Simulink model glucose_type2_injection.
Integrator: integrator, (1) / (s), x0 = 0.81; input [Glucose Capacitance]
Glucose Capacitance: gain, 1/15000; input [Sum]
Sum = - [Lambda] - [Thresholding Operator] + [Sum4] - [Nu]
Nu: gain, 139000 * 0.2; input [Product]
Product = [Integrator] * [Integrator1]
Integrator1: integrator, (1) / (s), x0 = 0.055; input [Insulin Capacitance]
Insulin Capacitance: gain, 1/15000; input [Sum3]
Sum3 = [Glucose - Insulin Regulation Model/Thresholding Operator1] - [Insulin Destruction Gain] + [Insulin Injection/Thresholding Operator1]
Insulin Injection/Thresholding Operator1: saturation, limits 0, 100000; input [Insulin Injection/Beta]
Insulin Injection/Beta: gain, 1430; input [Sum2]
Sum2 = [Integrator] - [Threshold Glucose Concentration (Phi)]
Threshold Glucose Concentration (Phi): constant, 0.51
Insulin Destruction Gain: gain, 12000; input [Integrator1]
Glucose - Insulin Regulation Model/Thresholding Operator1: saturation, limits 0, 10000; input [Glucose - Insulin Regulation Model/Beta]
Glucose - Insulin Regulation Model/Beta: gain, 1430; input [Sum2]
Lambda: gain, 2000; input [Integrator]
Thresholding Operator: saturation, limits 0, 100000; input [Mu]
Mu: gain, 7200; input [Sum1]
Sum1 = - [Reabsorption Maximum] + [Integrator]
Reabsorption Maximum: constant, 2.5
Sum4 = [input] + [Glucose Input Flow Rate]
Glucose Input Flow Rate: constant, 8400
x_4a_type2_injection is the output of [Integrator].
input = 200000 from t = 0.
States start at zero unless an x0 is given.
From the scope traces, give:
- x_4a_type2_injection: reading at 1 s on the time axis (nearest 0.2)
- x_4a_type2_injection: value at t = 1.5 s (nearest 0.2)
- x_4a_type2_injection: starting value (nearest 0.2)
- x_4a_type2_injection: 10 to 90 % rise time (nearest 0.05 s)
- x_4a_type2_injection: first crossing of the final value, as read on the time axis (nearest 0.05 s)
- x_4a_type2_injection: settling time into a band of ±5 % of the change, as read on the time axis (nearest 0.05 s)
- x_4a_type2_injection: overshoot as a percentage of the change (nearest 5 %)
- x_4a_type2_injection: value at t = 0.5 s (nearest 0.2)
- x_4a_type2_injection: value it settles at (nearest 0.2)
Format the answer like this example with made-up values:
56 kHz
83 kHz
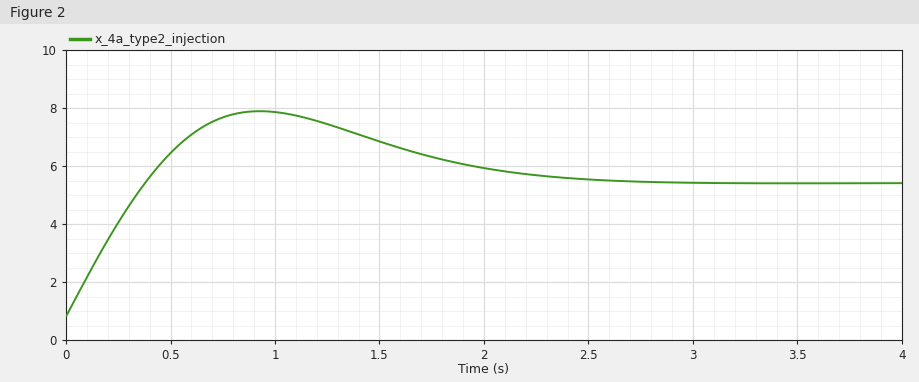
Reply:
7.8
6.8
0.8
0.30 s
0.40 s
2.30 s
55 %
6.4
5.4
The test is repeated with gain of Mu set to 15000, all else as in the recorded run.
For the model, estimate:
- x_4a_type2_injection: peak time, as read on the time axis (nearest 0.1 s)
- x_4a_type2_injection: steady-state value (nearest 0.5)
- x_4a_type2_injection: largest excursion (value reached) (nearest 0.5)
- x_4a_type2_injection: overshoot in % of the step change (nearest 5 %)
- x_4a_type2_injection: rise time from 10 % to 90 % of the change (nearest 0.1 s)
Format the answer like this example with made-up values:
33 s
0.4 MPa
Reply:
0.9 s
5.0
7.0
45 %
0.3 s
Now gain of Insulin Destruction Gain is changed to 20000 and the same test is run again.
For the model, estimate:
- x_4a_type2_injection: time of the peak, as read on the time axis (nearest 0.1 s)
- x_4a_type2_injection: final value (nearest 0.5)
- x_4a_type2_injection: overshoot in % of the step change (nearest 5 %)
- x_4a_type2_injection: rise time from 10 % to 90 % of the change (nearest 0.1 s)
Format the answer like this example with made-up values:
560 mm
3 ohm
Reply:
1.0 s
6.5
25 %
0.4 s
